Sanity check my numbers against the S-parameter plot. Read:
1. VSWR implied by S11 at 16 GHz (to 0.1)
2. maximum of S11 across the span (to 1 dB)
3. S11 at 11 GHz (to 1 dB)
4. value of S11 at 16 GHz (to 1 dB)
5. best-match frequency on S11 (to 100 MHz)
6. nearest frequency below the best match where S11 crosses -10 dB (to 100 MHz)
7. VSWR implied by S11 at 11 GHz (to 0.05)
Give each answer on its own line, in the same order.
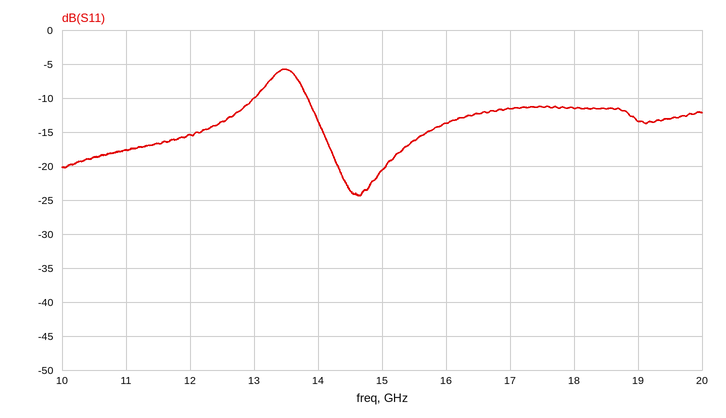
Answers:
1.5
-6 dB
-18 dB
-14 dB
14.6 GHz
13.8 GHz
1.30
